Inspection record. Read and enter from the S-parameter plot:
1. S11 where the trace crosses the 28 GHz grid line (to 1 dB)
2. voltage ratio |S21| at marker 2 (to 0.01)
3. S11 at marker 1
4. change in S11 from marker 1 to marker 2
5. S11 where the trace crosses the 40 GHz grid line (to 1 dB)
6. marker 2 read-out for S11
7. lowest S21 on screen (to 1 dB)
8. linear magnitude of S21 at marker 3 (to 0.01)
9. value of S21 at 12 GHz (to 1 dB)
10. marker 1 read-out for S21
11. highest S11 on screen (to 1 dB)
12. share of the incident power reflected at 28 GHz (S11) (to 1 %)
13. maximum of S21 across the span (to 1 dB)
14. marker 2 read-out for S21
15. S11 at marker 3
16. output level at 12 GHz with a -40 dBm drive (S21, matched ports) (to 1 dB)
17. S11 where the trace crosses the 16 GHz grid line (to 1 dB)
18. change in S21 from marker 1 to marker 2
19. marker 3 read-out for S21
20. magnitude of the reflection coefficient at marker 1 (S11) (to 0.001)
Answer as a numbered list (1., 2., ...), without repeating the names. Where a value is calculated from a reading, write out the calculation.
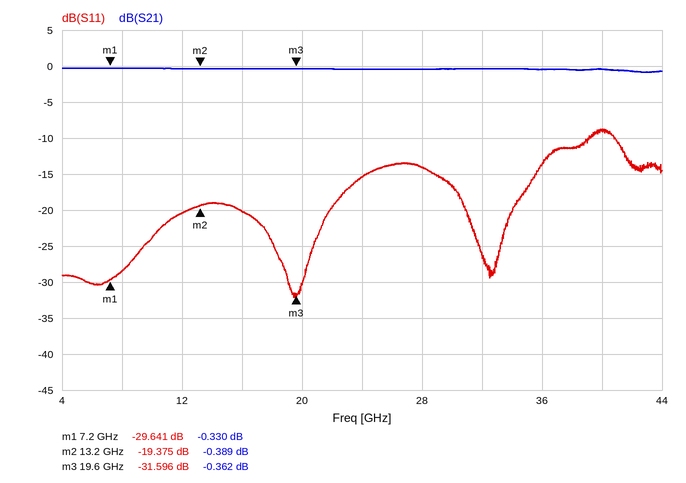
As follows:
1. -14 dB
2. 10^(-0.389/20) ≈ 0.96
3. -29.641 dB
4. -19.375 − (-29.641) = 10.266 dB
5. -9 dB
6. -19.375 dB
7. -1 dB
8. 10^(-0.362/20) ≈ 0.96
9. 0 dB
10. -0.330 dB
11. -9 dB
12. 10^(-14/10) ≈ 4 %
13. 0 dB
14. -0.389 dB
15. -31.596 dB
16. -40 dBm + (0 dB) = -40 dBm
17. -20 dB
18. -0.389 − (-0.33) = -0.059 dB
19. -0.362 dB
20. 10^(-29.641/20) ≈ 0.033
